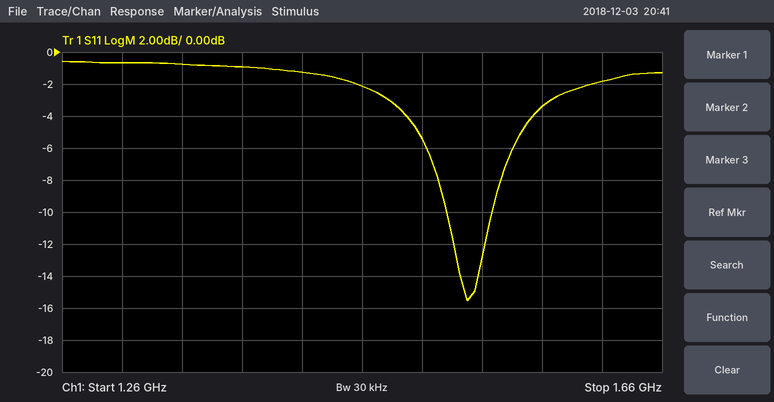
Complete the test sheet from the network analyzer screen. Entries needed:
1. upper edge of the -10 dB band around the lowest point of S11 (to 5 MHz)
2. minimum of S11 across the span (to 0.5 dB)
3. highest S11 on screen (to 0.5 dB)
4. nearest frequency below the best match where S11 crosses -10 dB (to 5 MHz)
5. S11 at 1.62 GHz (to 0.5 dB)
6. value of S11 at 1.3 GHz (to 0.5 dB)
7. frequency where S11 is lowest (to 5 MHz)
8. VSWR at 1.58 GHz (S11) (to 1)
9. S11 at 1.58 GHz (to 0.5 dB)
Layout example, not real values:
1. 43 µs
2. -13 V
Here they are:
1. 1.545 GHz
2. -15.5 dB
3. -0.5 dB
4. 1.515 GHz
5. -2.0 dB
6. -0.5 dB
7. 1.530 GHz
8. 5
9. -3.5 dB
